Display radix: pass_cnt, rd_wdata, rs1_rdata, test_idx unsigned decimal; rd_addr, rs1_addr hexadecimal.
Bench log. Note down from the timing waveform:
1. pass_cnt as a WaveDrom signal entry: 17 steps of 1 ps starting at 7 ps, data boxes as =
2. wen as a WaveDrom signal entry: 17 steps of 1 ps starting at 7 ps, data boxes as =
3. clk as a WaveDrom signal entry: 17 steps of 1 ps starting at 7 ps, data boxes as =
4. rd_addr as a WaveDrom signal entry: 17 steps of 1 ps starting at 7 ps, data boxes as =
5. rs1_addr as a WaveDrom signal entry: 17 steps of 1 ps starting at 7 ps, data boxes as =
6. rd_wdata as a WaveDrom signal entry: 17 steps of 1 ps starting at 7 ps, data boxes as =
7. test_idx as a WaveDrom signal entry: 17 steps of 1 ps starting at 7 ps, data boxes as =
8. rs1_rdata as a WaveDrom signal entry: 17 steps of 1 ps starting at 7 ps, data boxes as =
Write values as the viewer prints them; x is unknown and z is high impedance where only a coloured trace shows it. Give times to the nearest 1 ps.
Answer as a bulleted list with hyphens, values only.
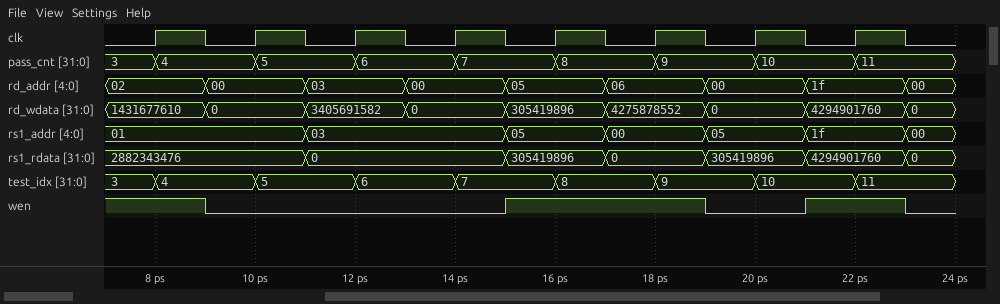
- {name: 'pass_cnt', wave: '==.=.=.=.=.=.=.=.', data: '3 4 5 6 7 8 9 10 11'}
- {name: 'wen', wave: '1.0.....1...0.1.0'}
- {name: 'clk', wave: '01010101010101010'}
- {name: 'rd_addr', wave: '=.=.=.=.=.=.=.=.=', data: '02 00 03 00 05 06 00 1f 00'}
- {name: 'rs1_addr', wave: '=...=...=.=.=.=.=', data: '01 03 05 00 05 1f 00'}
- {name: 'rd_wdata', wave: '=.=.=.=.=.=.=.=.=', data: '1431677610 0 3405691582 0 305419896 4275878552 0 4294901760 0'}
- {name: 'test_idx', wave: '==.=.=.=.=.=.=.=.', data: '3 4 5 6 7 8 9 10 11'}
- {name: 'rs1_rdata', wave: '=...=...=.=.=.=.=', data: '2882343476 0 305419896 0 305419896 4294901760 0'}
